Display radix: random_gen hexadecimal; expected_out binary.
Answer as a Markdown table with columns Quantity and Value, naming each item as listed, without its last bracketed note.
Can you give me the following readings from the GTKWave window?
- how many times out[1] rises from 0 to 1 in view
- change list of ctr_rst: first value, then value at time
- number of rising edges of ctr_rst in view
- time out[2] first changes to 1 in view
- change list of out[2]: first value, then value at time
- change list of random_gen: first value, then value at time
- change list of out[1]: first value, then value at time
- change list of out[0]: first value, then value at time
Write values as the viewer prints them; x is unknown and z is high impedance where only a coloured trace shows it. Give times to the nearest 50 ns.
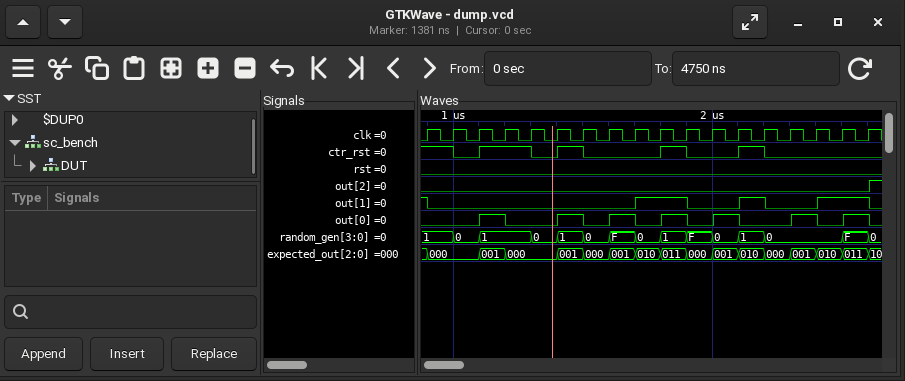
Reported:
| Quantity | Value |
|---|---|
| how many times out[1] rises from 0 to 1 in view | 3 |
| change list of ctr_rst: first value, then value at time | 1, 0 at 1000 ns, 1 at 1100 ns, 0 at 1300 ns, 1 at 1400 ns, 0 at 1500 ns, 1 at 1800 ns, 0 at 1900 ns, 1 at 2100 ns, 0 at 2200 ns |
| number of rising edges of ctr_rst in view | 4 |
| time out[2] first changes to 1 in view | 2600 ns |
| change list of out[2]: first value, then value at time | 0, 1 at 2600 ns |
| change list of random_gen: first value, then value at time | 1, 0 at 1000 ns, 1 at 1100 ns, 0 at 1300 ns, 1 at 1400 ns, 0 at 1500 ns, F at 1600 ns, 0 at 1700 ns, 1 at 1800 ns, F at 1900 ns, 0 at 2000 ns, 1 at 2100 ns, 0 at 2200 ns, F at 2500 ns, 0 at 2600 ns |
| change list of out[1]: first value, then value at time | 1, 0 at 900 ns, 1 at 1700 ns, 0 at 1900 ns, 1 at 2100 ns, 0 at 2200 ns, 1 at 2400 ns, 0 at 2600 ns |
| change list of out[0]: first value, then value at time | 0, 1 at 1100 ns, 0 at 1200 ns, 1 at 1400 ns, 0 at 1500 ns, 1 at 1600 ns, 0 at 1700 ns, 1 at 1800 ns, 0 at 1900 ns, 1 at 2000 ns, 0 at 2100 ns, 1 at 2300 ns, 0 at 2400 ns, 1 at 2500 ns, 0 at 2600 ns |
